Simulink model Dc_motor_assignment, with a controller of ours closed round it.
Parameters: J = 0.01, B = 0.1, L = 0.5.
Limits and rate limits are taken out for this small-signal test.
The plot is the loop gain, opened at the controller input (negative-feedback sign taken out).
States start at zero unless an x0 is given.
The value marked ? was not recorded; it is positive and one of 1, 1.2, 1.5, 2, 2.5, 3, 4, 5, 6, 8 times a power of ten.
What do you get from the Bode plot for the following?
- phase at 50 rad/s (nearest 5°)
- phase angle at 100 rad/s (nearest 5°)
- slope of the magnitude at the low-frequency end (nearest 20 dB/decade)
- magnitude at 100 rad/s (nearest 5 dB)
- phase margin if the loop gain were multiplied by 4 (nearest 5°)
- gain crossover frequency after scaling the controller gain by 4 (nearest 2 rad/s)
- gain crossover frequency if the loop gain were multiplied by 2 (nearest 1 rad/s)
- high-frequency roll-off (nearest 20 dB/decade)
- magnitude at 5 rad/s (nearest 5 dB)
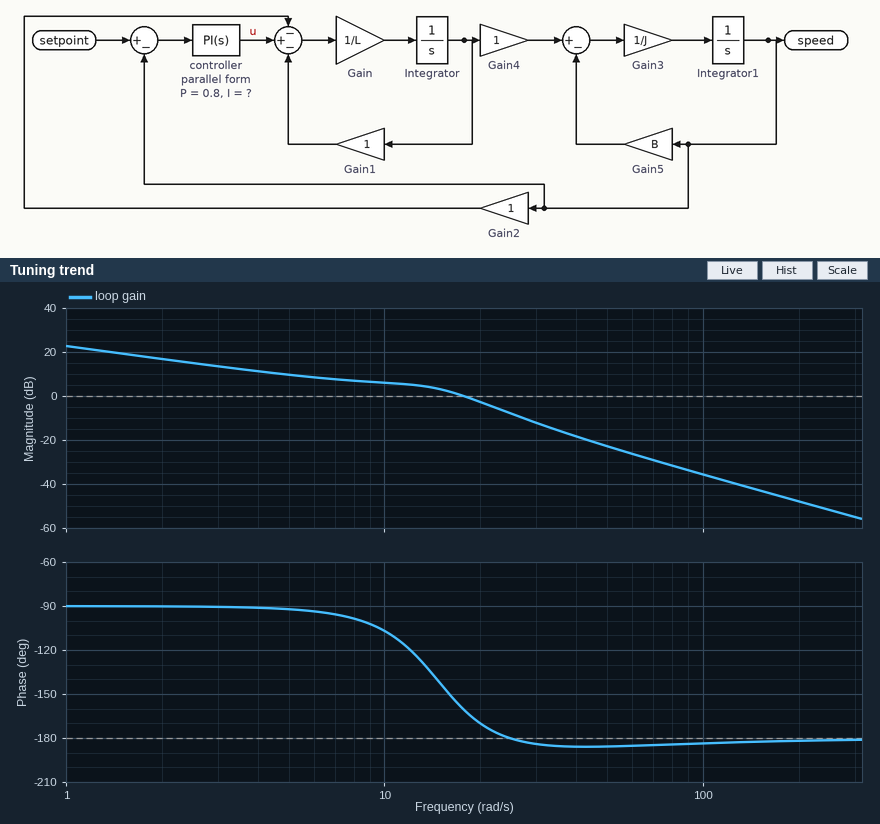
-185°
-185°
-20 dB/decade
-35 dB
-5°
30 rad/s
23 rad/s
-40 dB/decade
10 dB
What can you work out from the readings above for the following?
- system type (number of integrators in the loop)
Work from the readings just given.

1
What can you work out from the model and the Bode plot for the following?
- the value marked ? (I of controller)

15
